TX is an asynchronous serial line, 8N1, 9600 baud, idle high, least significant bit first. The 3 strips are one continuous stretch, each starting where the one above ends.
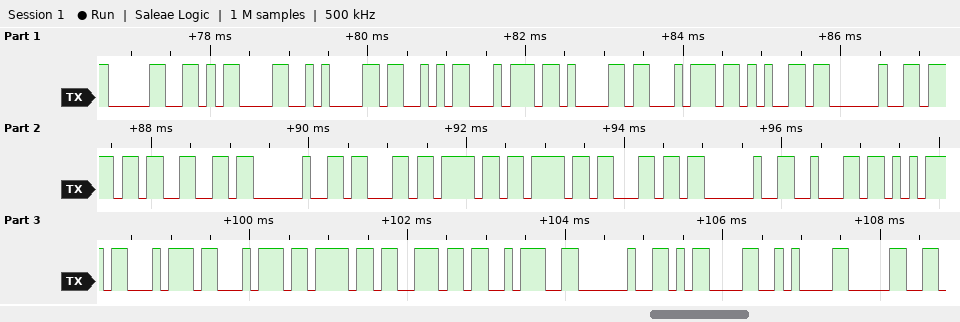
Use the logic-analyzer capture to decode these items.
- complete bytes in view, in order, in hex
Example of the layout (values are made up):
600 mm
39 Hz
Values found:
30 0D 0A 53 74 61 74 65 20 6F 66 20 63 6F 6F 6C 20 62 75 74 74 6F 6E 3A 20 0D 0A 30
